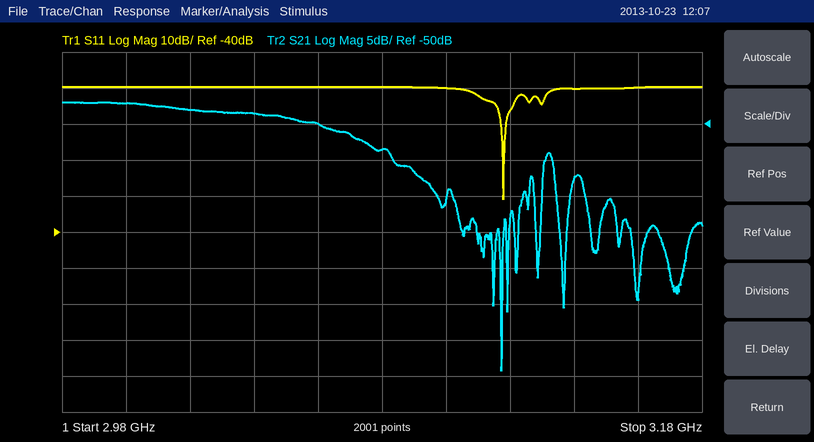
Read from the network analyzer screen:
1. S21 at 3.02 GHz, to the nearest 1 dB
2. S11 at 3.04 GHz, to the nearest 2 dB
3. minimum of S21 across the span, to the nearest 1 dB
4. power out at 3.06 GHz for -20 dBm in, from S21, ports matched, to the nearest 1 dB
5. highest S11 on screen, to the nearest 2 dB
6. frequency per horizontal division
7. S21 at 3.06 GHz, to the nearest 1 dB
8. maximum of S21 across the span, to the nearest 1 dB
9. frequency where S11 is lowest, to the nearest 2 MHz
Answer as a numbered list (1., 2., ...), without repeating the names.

1. -48 dB
2. 0 dB
3. -84 dB
4. -70 dBm
5. 0 dB
6. 20 MHz
7. -50 dB
8. -47 dB
9. 3.118 GHz
